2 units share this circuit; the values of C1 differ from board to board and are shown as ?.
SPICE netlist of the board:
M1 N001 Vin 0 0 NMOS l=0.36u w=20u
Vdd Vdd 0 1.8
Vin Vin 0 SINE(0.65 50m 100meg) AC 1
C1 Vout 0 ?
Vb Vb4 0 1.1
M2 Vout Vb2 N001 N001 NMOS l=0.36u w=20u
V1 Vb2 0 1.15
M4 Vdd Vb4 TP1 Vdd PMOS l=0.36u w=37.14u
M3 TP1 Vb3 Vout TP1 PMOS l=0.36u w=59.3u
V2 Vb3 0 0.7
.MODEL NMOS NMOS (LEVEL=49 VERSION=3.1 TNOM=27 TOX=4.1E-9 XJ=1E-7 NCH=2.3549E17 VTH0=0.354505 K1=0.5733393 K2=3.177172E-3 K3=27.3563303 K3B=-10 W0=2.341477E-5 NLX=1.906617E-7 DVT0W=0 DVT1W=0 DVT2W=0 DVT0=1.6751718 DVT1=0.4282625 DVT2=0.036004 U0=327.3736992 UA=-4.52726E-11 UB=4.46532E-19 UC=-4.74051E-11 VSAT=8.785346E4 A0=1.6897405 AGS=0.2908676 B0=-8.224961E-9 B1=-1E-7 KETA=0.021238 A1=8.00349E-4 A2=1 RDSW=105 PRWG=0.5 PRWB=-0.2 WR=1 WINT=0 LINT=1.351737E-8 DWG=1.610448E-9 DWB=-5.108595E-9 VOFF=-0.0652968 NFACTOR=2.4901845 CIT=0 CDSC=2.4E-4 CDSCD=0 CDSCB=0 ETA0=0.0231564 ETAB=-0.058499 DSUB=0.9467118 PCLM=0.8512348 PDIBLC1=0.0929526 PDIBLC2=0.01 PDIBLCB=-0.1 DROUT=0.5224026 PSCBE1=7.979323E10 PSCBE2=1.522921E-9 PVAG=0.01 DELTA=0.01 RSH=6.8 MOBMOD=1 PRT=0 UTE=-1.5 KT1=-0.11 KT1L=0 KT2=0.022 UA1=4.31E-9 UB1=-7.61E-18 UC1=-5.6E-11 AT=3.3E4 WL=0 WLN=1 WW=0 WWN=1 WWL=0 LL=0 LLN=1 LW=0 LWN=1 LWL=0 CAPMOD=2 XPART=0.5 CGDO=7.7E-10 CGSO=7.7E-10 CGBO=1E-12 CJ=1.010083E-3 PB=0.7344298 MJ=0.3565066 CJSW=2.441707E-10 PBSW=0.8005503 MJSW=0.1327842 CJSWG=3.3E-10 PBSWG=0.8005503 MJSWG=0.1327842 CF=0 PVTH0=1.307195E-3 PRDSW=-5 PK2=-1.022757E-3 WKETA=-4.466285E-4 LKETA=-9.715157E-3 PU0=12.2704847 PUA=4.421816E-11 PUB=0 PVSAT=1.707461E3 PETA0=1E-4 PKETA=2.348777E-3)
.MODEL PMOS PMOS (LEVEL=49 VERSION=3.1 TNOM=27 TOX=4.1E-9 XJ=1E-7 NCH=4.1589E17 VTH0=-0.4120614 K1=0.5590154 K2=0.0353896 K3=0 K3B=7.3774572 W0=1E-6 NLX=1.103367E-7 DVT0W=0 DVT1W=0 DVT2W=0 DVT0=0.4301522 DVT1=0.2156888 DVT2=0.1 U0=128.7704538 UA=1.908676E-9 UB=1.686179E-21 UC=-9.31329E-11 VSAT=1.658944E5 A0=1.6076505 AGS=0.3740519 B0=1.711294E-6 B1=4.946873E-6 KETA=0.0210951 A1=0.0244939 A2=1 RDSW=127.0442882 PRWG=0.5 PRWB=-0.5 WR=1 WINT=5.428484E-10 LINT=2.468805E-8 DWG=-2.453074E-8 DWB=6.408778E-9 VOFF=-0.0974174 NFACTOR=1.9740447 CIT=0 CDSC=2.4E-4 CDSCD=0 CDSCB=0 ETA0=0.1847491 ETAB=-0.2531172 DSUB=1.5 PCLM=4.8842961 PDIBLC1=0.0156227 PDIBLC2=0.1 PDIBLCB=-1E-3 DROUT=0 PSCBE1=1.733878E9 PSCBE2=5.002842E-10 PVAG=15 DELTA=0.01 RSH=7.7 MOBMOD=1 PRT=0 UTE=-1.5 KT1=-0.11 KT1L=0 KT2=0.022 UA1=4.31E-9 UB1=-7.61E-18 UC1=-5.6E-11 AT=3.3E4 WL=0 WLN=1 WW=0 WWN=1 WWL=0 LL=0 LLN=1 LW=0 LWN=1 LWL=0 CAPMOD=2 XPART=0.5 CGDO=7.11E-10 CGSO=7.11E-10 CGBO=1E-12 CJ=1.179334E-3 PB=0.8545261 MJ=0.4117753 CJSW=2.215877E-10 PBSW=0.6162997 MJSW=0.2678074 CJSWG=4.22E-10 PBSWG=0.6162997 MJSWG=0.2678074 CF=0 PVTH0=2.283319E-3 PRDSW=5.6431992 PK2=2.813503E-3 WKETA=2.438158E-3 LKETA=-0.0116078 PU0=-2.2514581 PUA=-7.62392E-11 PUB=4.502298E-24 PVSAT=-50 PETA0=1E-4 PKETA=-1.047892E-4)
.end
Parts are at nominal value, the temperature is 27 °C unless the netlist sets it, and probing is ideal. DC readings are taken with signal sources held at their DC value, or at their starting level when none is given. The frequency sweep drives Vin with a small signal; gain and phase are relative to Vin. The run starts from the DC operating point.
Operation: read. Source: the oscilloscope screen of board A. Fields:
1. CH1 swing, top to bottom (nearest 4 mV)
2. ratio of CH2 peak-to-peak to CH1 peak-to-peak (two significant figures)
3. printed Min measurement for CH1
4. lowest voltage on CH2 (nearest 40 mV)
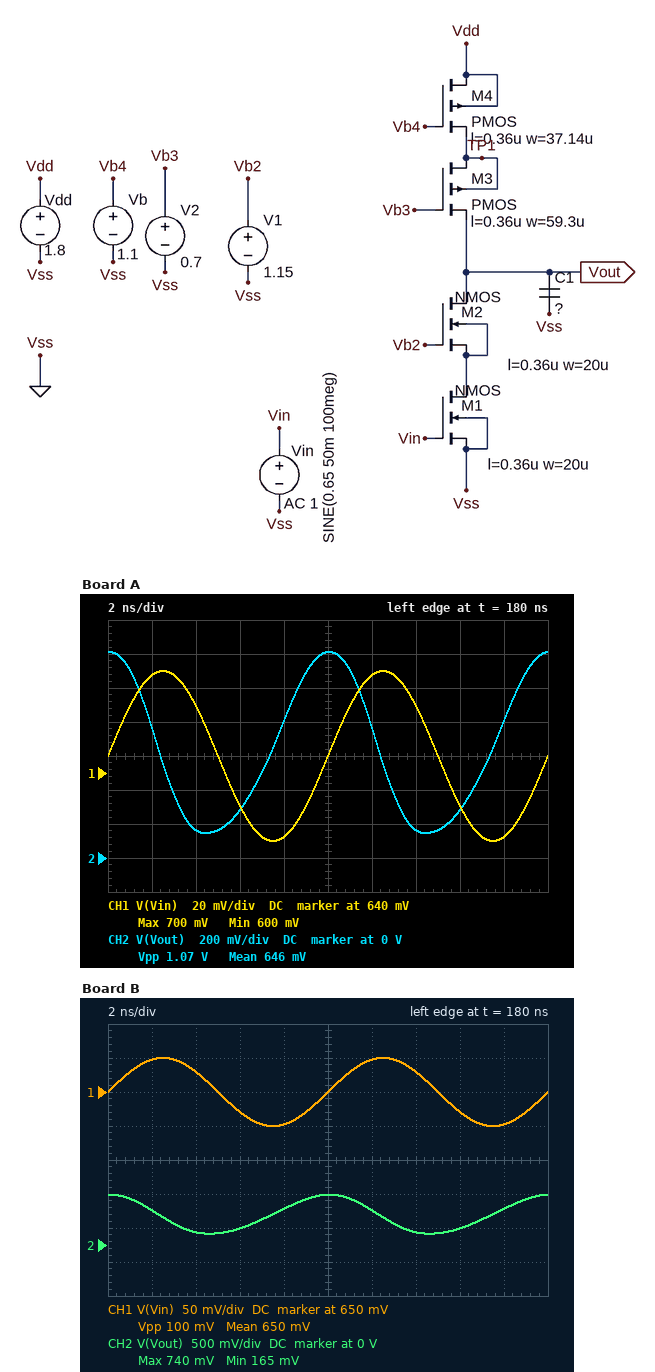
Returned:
100 mV
11
600 mV
160 mV
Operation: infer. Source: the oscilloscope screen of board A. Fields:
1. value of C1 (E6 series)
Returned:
220 fF
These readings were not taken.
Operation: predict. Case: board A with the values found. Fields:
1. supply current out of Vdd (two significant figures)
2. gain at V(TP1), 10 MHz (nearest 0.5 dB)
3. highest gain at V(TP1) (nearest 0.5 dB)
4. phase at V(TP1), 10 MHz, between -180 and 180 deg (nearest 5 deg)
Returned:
190 µA
32.0 dB
41.0 dB
110 deg
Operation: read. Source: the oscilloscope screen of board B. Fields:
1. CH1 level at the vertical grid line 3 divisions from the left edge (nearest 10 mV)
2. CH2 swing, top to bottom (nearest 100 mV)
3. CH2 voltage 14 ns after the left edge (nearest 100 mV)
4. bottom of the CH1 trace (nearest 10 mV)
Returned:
620 mV
600 mV
200 mV
600 mV
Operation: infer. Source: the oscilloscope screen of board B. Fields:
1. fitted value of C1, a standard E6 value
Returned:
470 fF
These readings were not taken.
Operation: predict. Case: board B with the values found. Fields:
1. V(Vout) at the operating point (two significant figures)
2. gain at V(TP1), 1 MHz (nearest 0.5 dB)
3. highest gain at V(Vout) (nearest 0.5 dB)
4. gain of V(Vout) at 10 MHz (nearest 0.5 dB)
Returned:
1.3 V
40.0 dB
47.0 dB
34.5 dB
